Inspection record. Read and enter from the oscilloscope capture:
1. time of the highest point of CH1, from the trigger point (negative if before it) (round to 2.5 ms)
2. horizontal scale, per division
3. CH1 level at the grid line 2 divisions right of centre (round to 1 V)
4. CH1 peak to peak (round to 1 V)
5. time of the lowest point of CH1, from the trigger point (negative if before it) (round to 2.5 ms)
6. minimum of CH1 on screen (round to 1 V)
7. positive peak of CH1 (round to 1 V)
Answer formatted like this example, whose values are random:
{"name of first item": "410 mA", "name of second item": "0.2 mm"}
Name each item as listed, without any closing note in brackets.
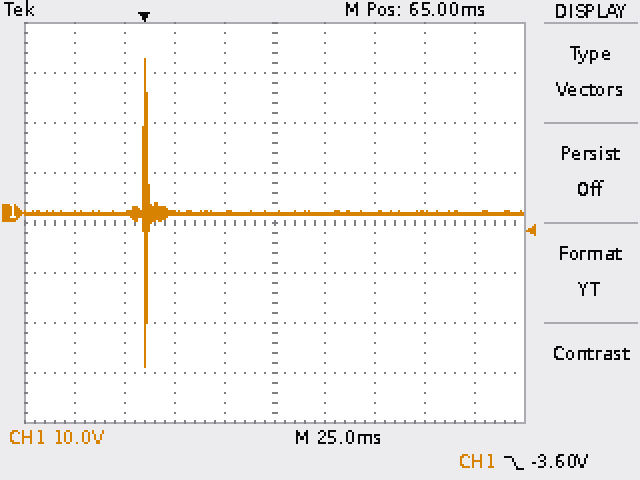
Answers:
{"time of the highest point of CH1, from the trigger point (negative if before it)": "0.0 ms", "horizontal scale, per division": "25 ms", "CH1 level at the grid line 2 divisions right of centre": "0 V", "CH1 peak to peak": "62 V", "time of the lowest point of CH1, from the trigger point (negative if before it)": "0.0 ms", "minimum of CH1 on screen": "-31 V", "positive peak of CH1": "31 V"}
